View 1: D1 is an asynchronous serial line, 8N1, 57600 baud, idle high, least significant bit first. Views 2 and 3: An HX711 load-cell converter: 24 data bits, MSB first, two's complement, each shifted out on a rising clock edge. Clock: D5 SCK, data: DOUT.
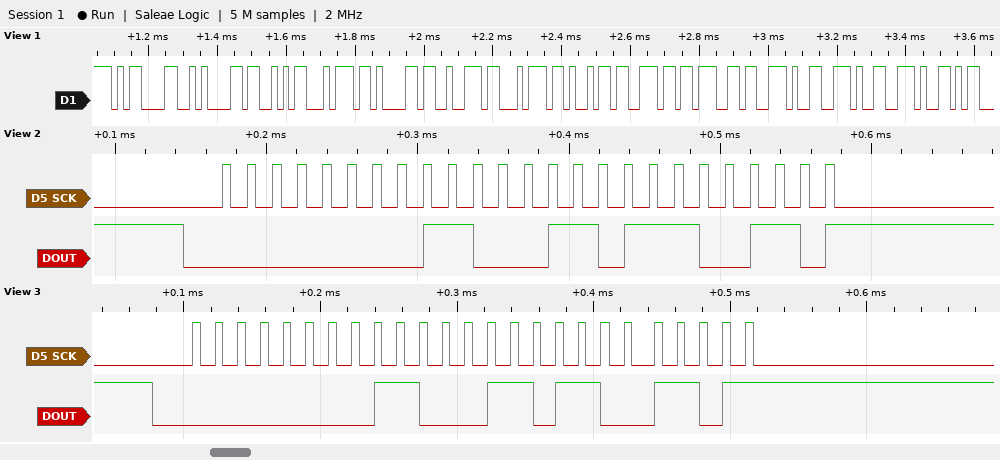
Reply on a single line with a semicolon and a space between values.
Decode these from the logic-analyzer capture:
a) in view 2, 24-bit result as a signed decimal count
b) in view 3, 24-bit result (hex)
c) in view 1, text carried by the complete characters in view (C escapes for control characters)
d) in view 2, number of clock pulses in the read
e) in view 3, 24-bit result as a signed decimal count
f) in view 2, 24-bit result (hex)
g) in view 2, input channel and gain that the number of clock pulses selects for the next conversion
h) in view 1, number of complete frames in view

50918; 0x00C6CD; "\r\nStarting..."; 25; 50893; 0x00C6E6; channel A, gain 128; 13
